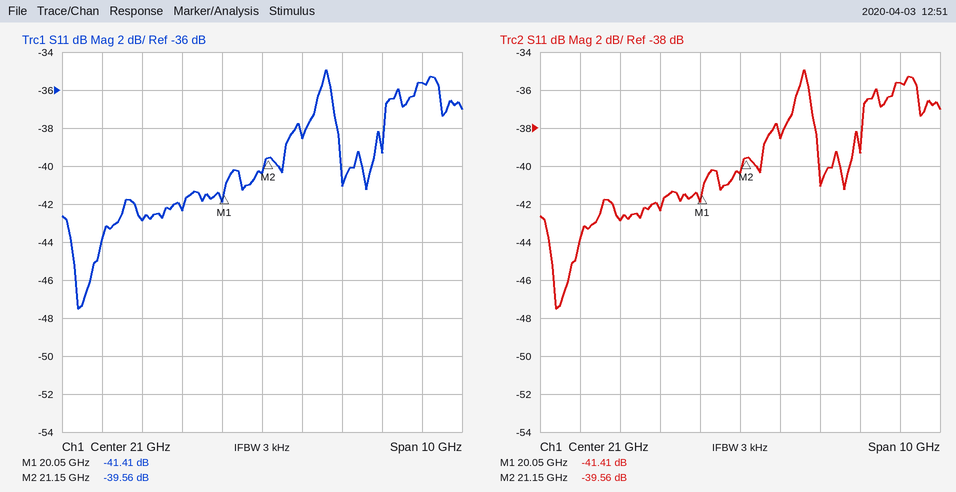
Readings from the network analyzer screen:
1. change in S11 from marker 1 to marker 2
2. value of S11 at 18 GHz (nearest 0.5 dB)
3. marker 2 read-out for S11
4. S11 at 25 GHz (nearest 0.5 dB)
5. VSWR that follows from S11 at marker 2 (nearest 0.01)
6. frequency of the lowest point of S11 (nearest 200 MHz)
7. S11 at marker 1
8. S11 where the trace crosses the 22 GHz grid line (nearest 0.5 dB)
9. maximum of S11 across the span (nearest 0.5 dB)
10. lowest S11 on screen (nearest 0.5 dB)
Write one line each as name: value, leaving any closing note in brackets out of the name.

change in S11 from marker 1 to marker 2: 1.85 dB
value of S11 at 18 GHz: -43.0 dB
marker 2 read-out for S11: -39.56 dB
S11 at 25 GHz: -35.5 dB
VSWR that follows from S11 at marker 2: 1.02
frequency of the lowest point of S11: 16.4 GHz
S11 at marker 1: -41.41 dB
S11 where the trace crosses the 22 GHz grid line: -38.5 dB
maximum of S11 across the span: -35.0 dB
lowest S11 on screen: -47.5 dB
